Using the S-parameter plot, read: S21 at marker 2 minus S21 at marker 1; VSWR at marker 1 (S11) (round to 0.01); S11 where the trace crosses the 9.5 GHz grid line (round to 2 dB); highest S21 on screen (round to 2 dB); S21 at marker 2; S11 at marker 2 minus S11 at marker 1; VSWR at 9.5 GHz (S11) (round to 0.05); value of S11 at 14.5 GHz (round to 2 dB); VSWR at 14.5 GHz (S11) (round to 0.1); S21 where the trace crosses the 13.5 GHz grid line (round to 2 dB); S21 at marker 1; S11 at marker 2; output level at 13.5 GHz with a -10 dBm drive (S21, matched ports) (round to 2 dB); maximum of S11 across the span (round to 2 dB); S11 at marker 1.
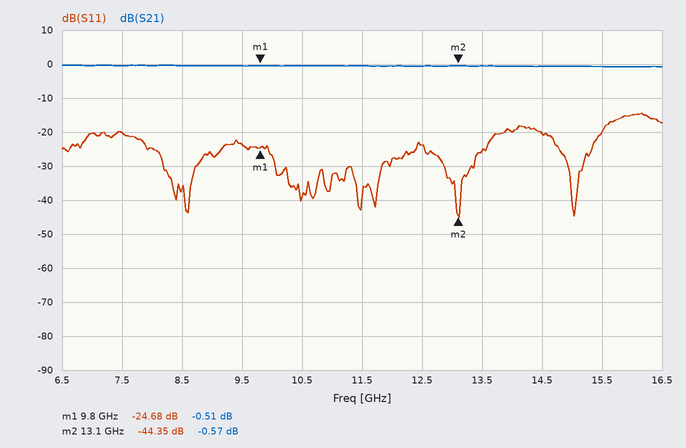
-0.06 dB
1.12
-24 dB
0 dB
-0.57 dB
-19.67 dB
1.15
-20 dB
1.2
0 dB
-0.51 dB
-44.35 dB
-10 dBm
-14 dB
-24.68 dB
